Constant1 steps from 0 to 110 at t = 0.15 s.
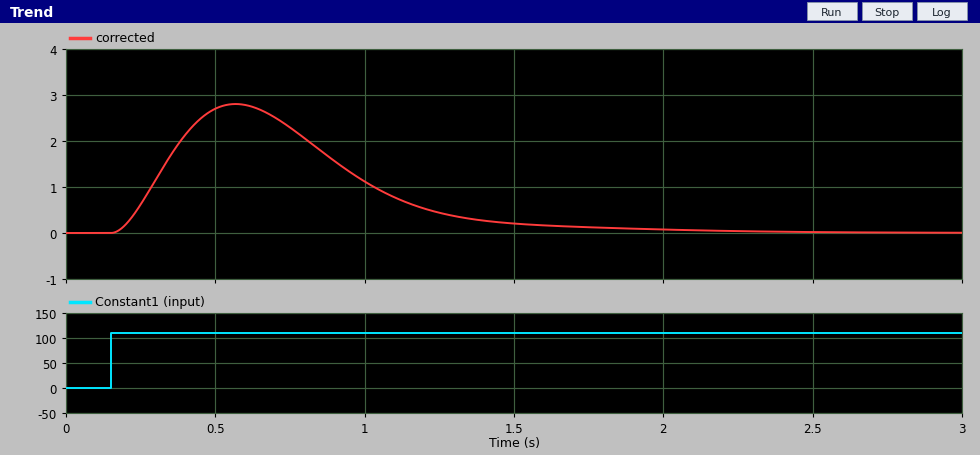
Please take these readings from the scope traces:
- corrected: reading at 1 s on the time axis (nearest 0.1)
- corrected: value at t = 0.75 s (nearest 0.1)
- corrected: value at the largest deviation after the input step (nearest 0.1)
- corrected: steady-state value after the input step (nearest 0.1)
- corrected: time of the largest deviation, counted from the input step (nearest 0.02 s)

1.1
2.3
2.8
0.0
0.42 s
